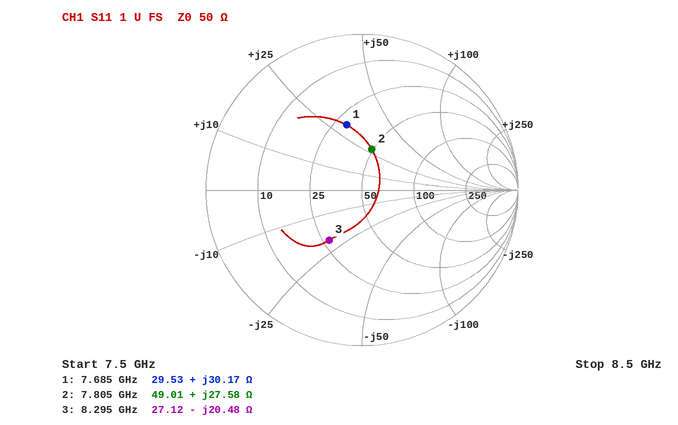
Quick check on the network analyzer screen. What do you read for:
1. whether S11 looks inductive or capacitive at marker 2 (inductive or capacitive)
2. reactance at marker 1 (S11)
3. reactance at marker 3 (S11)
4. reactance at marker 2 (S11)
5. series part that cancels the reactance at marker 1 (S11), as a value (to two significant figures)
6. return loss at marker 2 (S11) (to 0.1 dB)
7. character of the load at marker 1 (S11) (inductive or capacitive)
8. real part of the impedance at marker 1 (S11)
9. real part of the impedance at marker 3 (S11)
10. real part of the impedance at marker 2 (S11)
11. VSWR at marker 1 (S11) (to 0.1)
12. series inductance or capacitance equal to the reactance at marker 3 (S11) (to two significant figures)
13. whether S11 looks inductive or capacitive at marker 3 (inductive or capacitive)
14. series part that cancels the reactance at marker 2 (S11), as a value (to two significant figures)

inductive
+30.17 Ω
-20.48 Ω
+27.58 Ω
690 fF
11.4 dB
inductive
29.53 Ω
27.12 Ω
49.01 Ω
2.5
940 fF
capacitive
740 fF
